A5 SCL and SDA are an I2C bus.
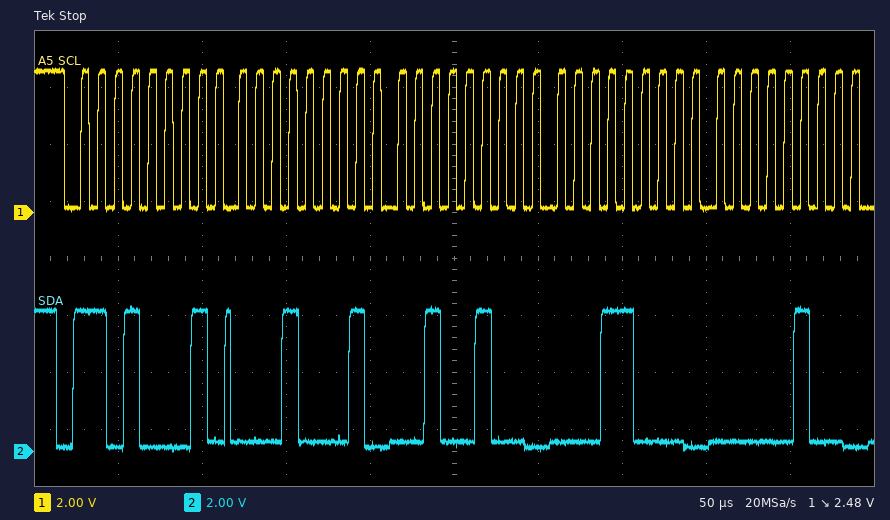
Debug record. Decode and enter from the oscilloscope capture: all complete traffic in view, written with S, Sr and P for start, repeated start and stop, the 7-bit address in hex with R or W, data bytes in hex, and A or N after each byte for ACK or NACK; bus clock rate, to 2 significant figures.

S 68R A 11 A 24 A 18 A 04 A
100 kHz
